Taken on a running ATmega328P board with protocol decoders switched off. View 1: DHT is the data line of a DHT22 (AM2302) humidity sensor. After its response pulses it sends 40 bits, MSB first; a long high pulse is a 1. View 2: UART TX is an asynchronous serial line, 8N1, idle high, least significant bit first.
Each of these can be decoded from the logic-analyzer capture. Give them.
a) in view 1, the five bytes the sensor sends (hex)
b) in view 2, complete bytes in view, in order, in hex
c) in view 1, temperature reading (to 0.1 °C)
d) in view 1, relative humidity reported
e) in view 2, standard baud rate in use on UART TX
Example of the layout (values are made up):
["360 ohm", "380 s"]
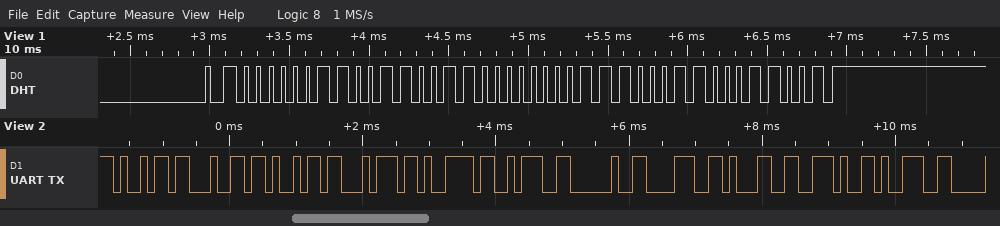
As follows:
["03 33 00 E3 19", "69 64 69 74 79 3A 20 38 31 2E 39", "22.7 °C", "81.9 %", "9600 baud"]
